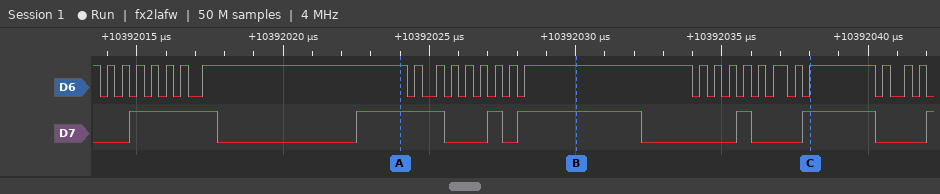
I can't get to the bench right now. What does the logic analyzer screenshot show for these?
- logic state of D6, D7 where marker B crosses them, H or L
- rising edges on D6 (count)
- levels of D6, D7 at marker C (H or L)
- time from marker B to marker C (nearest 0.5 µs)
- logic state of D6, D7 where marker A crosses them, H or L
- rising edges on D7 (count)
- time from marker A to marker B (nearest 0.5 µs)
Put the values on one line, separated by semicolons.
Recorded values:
D6=H, D7=H; 26; D6=H, D7=H; 8 µs; D6=H, D7=H; 7; 6 µs
